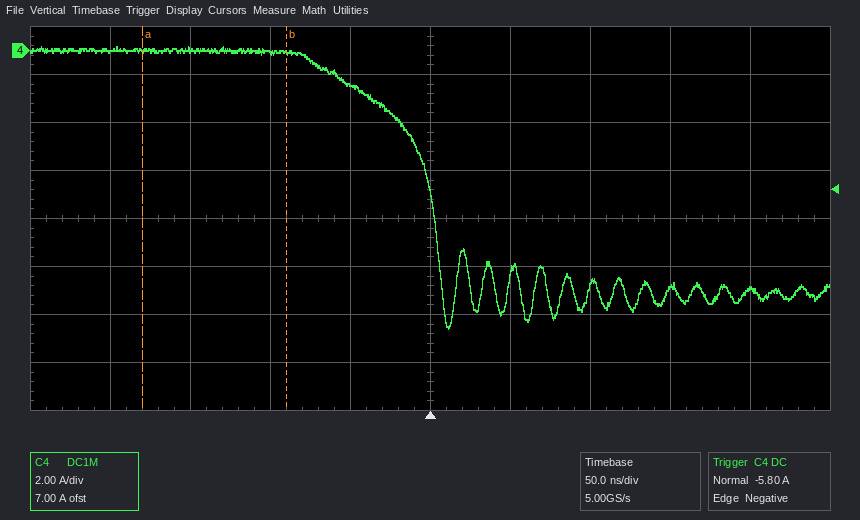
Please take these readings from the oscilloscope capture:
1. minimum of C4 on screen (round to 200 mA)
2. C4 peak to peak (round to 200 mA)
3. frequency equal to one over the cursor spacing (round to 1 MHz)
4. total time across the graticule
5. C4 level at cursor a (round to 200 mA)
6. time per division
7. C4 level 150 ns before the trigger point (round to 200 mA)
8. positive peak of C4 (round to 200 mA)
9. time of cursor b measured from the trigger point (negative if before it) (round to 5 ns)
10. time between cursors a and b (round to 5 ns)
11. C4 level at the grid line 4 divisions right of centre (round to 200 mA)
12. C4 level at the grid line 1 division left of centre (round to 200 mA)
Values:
-11.6 A
11.8 A
11 MHz
500 ns
0.0 A
50 ns
0.0 A
200 mA
-90 ns
90 ns
-10.0 A
-1.4 A
